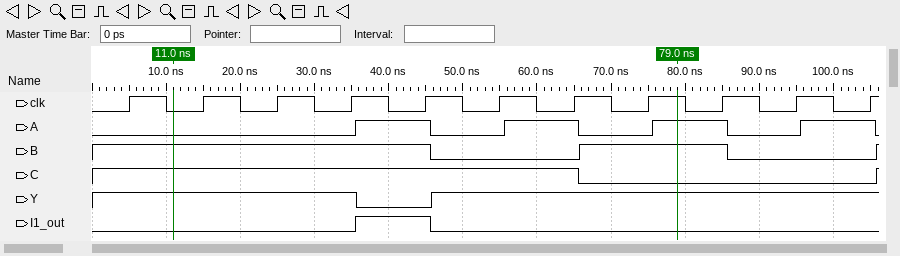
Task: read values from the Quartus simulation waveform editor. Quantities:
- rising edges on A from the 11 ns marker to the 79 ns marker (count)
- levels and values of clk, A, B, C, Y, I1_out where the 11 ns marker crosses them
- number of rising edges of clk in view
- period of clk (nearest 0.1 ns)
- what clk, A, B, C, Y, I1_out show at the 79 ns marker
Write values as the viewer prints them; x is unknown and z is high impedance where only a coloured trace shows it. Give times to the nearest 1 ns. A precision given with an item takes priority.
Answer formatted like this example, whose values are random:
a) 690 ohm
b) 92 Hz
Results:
a) 3
b) clk=0, A=0, B=1, C=1, Y=1, I1_out=0
c) 11
d) 10 ns
e) clk=1, A=1, B=1, C=0, Y=1, I1_out=0
